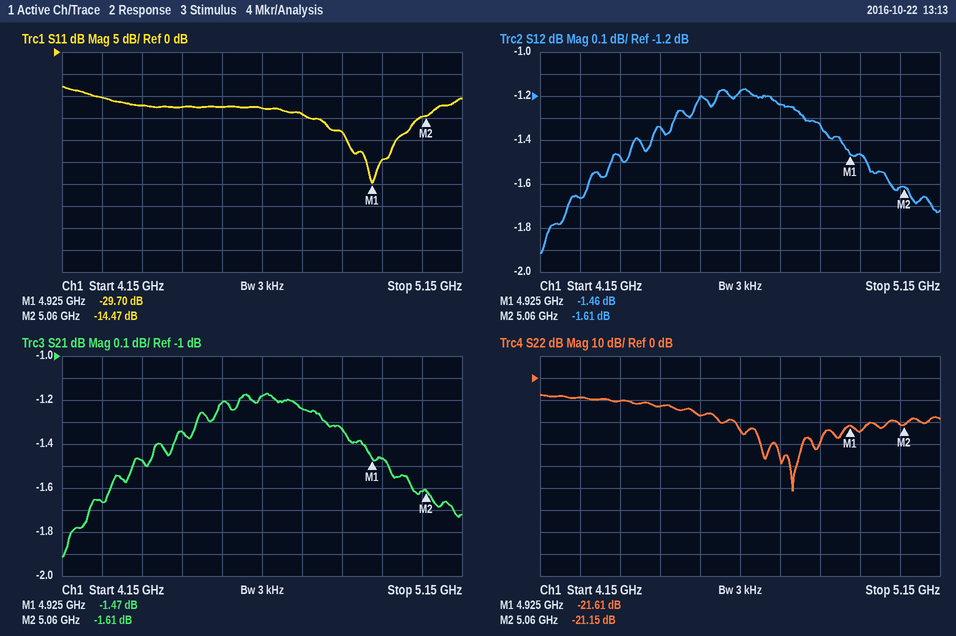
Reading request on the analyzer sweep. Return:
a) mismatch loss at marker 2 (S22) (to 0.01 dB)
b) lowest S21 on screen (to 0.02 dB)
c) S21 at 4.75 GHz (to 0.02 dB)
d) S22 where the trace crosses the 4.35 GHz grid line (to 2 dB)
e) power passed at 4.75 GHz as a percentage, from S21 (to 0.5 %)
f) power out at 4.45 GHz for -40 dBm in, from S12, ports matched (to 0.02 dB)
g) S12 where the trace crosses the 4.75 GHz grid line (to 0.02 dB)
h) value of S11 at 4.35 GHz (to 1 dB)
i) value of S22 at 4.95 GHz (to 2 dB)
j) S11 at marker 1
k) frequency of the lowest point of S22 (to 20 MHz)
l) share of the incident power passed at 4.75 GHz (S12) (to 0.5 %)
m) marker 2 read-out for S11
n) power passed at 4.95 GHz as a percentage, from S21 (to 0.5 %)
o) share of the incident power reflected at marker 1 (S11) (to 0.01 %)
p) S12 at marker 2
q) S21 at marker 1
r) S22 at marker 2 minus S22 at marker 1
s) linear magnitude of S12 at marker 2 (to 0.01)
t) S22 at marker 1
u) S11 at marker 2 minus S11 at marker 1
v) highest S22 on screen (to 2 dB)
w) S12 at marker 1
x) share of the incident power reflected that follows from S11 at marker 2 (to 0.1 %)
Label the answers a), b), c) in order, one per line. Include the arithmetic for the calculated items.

a) −10 log10(1 − 10^(-21.15/10)) ≈ 0.03 dB
b) -1.92 dB
c) -1.24 dB
d) -10 dB
e) 10^(-1.24/10) ≈ 75.2 %, so 75.0 % to the nearest 0.5 %
f) -40 dBm + (-1.34 dB) = -41.34 dBm
g) -1.24 dB
h) -12 dB
i) -24 dB
j) -29.70 dB
k) 4.78 GHz
l) 10^(-1.24/10) ≈ 75.2 %, so 75.0 % to the nearest 0.5 %
m) -14.47 dB
n) 10^(-1.46/10) ≈ 71.4 %, so 71.5 % to the nearest 0.5 %
o) 10^(-29.7/10) ≈ 0.11 %
p) -1.61 dB
q) -1.47 dB
r) -21.15 − (-21.61) = 0.46 dB
s) 10^(-1.61/20) ≈ 0.83
t) -21.61 dB
u) -14.47 − (-29.7) = 15.23 dB
v) -8 dB
w) -1.46 dB
x) 10^(-14.47/10) ≈ 3.6 %
